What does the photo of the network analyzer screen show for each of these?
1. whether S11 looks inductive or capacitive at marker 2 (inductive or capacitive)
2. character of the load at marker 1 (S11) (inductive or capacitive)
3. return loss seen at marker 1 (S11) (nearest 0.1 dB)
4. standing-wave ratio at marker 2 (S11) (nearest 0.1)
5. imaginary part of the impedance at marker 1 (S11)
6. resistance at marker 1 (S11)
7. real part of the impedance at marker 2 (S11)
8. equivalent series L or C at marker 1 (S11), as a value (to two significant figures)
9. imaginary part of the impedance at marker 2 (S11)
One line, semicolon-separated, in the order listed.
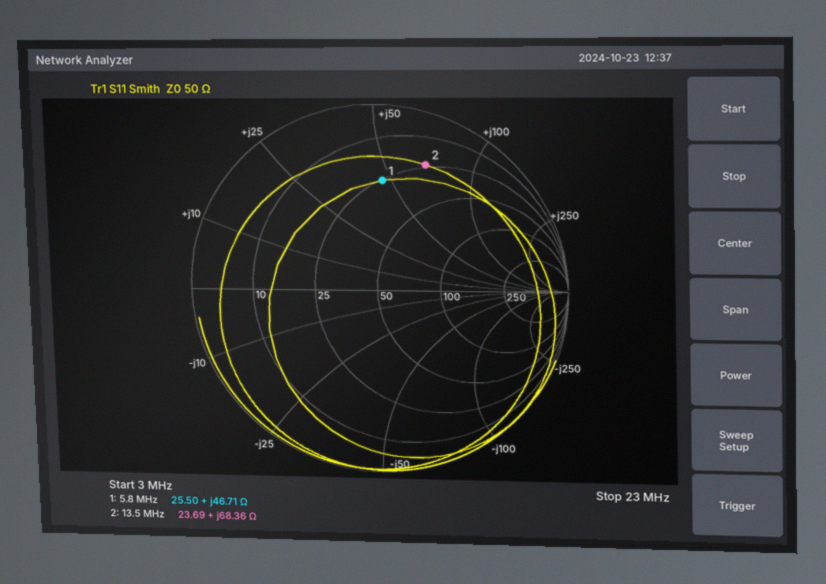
inductive; inductive; 4.5 dB; 6.4; +46.71 Ω; 25.50 Ω; 23.69 Ω; 1.3 µH; +68.36 Ω
